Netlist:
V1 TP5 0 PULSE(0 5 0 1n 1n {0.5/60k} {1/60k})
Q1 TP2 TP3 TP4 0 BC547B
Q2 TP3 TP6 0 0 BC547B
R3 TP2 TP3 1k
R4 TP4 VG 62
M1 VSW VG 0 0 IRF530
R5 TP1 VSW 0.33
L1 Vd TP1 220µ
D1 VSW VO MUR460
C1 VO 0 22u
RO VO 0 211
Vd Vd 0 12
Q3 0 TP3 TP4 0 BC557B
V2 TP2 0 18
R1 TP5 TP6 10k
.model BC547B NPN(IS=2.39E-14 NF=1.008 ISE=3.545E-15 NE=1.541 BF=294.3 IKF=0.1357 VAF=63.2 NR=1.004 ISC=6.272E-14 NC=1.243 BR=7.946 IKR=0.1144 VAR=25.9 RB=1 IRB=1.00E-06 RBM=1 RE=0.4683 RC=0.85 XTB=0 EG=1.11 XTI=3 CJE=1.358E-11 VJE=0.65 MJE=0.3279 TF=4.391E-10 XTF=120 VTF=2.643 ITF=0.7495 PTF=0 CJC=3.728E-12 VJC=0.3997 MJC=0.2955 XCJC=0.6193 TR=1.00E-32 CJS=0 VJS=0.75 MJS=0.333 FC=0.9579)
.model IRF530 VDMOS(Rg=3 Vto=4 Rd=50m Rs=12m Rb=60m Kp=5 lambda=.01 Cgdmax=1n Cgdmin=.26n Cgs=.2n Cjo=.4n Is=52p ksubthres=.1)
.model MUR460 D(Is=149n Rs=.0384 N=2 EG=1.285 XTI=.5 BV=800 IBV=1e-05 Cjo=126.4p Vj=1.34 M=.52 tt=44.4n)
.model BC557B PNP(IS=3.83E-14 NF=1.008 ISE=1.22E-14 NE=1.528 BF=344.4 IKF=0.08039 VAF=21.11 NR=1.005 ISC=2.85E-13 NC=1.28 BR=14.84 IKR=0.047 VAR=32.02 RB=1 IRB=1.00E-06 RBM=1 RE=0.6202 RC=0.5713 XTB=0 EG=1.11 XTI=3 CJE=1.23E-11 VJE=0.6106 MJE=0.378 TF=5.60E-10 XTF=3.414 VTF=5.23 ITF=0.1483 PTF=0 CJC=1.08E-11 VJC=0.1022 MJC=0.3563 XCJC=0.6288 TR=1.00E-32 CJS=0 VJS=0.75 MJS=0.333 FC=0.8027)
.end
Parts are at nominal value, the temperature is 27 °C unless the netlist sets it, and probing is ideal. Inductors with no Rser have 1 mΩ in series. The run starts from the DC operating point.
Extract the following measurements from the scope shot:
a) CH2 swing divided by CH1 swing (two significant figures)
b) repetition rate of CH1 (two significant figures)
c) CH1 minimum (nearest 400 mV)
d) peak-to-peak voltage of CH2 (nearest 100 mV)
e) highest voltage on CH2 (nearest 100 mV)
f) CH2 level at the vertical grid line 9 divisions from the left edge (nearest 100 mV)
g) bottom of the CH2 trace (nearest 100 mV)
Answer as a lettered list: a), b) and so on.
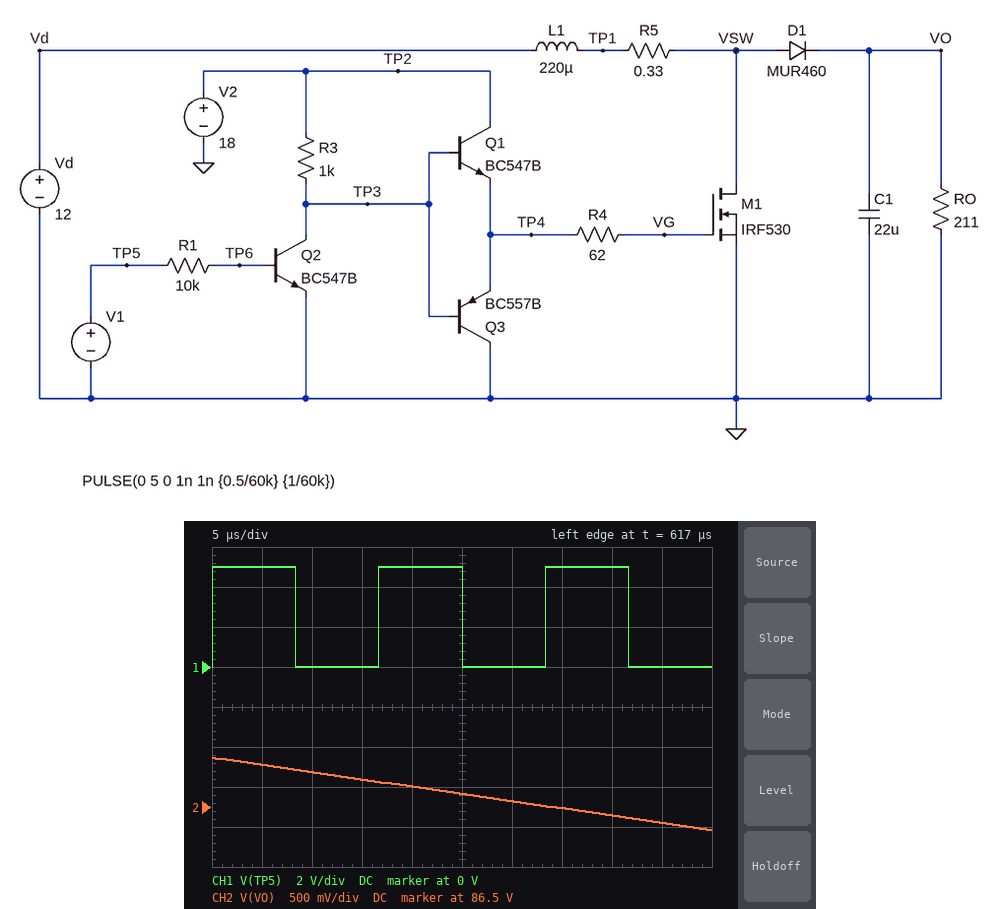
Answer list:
a) 0.18
b) 60 kHz
c) 0 V
d) 900 mV
e) 87.1 V
f) 86.3 V
g) 86.2 V
